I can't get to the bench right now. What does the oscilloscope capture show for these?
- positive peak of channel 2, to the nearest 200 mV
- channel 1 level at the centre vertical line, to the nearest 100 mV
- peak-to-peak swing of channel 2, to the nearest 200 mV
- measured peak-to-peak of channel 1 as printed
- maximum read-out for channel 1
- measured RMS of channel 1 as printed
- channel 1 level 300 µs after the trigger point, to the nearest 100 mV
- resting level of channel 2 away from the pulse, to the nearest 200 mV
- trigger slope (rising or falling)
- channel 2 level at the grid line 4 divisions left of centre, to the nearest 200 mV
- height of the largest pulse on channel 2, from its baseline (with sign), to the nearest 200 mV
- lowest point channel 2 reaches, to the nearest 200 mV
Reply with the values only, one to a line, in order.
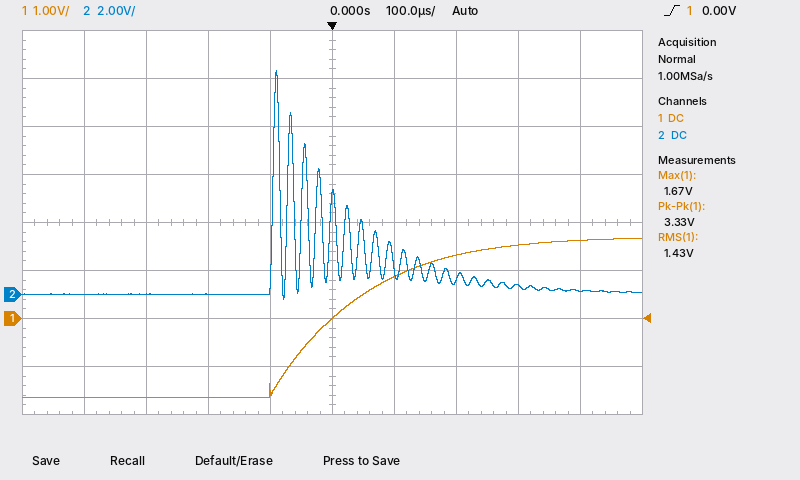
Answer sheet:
9.4 V
0.0 V
9.6 V
3.33 V
1.67 V
1.43 V
1.5 V
0.0 V
rising
0.0 V
+9.4 V
-200 mV
